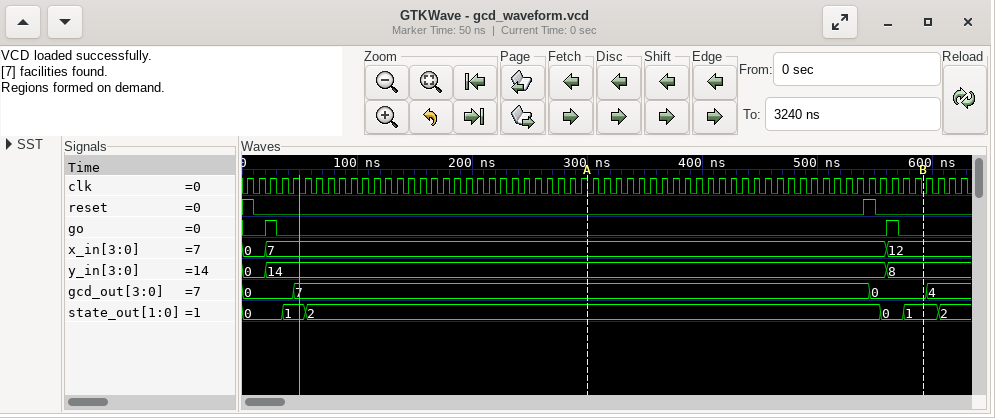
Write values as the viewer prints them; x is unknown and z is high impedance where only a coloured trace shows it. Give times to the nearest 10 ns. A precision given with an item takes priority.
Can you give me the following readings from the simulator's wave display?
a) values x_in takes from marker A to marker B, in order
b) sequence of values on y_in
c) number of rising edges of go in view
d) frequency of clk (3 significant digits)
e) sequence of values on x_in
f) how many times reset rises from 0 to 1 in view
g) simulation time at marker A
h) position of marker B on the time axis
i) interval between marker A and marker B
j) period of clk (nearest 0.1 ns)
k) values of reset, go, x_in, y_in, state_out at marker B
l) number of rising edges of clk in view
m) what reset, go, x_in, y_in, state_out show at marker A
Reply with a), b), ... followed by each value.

a) 7, 12
b) 0, 14, 8
c) 2
d) 100 MHz
e) 0, 7, 12
f) 1
g) 300 ns
h) 590 ns
i) 290 ns
j) 10 ns
k) reset=0, go=0, x_in=12, y_in=8, state_out=1
l) 63
m) reset=0, go=0, x_in=7, y_in=14, state_out=2
